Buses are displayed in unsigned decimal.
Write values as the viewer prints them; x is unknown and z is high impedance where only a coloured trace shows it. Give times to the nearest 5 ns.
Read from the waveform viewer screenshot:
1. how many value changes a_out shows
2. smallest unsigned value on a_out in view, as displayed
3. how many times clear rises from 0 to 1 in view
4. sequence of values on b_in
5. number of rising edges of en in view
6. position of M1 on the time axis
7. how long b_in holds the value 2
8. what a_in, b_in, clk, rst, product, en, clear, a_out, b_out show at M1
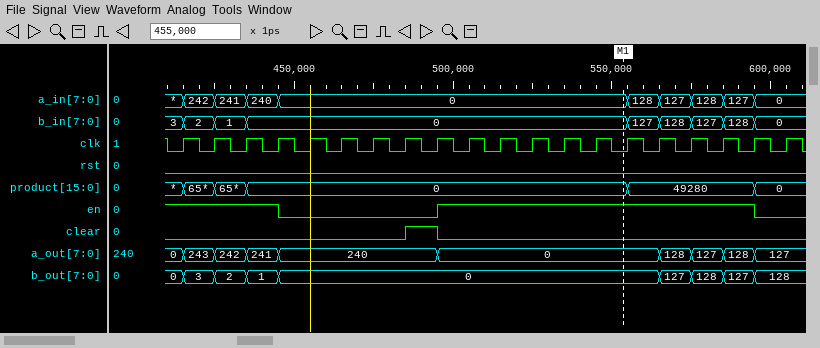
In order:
9
0
1
3, 2, 1, 0, 127, 128, 127, 128, 0
1
555 ns
10 ns
a_in=0, b_in=0, clk=0, rst=0, product=0, en=1, clear=0, a_out=0, b_out=0
